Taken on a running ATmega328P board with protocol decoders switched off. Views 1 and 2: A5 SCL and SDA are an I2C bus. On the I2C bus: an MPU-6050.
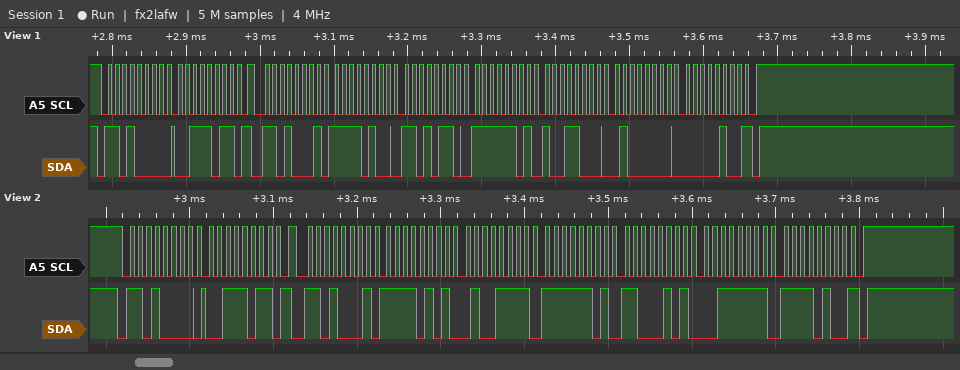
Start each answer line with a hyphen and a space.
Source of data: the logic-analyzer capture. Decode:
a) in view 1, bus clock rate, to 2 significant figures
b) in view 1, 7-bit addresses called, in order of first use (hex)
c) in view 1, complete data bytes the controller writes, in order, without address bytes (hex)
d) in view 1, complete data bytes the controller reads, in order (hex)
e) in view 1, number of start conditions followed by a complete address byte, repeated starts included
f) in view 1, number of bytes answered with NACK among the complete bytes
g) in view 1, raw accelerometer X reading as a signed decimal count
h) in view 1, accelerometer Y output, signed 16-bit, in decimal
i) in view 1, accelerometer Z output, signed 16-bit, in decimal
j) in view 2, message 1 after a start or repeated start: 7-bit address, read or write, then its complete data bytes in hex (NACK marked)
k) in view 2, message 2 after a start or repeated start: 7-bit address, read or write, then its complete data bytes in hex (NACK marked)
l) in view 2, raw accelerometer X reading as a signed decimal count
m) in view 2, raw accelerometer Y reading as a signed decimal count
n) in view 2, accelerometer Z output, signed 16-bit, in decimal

- 100 kHz
- 0x68
- 3B
- F4 D6 FD 98 40 04
- 2
- 1
- -2858
- -616
- 16388
- 0x68 write: 3B
- 0x68 read: F5 4F FD C5 3F F4 NACK
- -2737
- -571
- 16372
